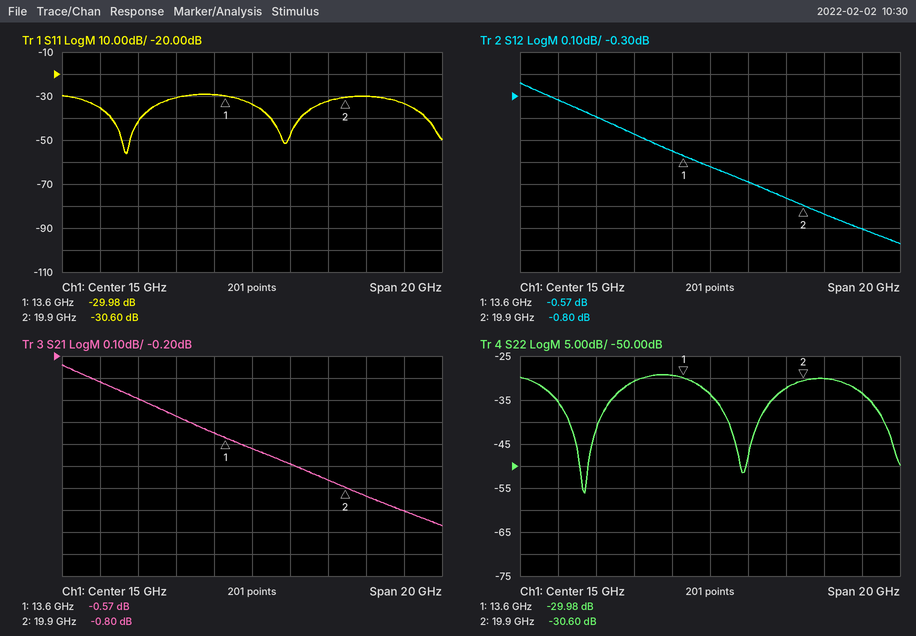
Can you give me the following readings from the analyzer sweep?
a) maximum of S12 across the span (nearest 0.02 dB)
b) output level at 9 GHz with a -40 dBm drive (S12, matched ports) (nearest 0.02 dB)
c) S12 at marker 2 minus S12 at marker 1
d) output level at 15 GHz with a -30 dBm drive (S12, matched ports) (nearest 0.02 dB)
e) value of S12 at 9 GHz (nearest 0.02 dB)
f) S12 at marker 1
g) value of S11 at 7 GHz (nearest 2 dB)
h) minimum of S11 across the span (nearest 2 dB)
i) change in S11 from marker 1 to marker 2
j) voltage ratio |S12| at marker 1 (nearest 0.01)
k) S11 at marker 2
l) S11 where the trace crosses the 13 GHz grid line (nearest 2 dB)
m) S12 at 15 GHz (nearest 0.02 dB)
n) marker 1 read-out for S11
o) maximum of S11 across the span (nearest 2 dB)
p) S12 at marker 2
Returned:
-0.24 dB
-40.40 dBm
-0.23 dB
-30.62 dBm
-0.40 dB
-0.57 dB
-36 dB
-56 dB
-0.62 dB
0.94
-30.60 dB
-30 dB
-0.62 dB
-29.98 dB
-30 dB
-0.80 dB
